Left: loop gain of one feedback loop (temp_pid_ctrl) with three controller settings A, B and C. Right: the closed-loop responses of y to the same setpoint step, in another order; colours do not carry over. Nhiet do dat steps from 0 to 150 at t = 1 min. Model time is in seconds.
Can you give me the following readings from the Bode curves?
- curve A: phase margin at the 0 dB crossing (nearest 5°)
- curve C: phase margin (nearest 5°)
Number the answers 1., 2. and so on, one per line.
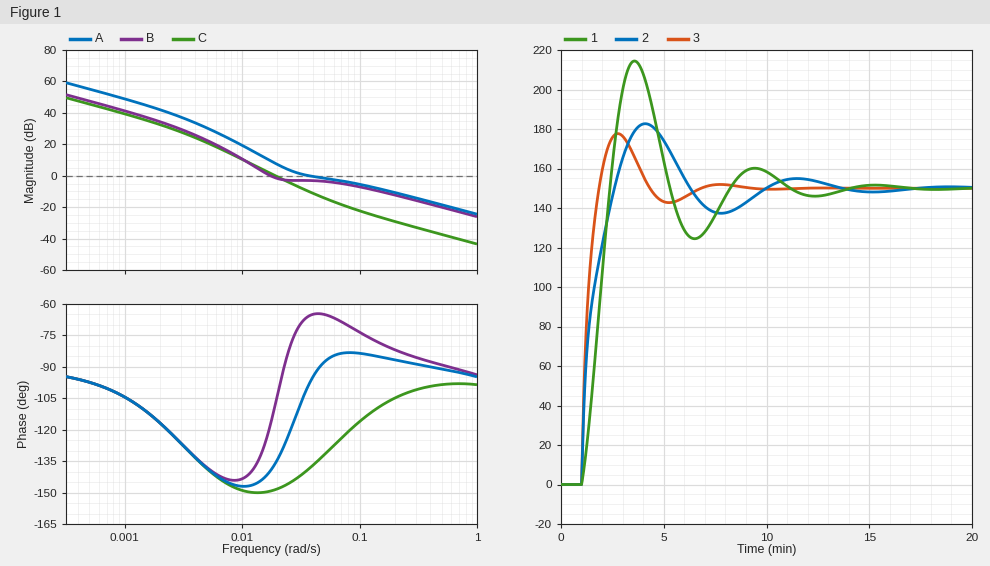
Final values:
1. 80°
2. 30°
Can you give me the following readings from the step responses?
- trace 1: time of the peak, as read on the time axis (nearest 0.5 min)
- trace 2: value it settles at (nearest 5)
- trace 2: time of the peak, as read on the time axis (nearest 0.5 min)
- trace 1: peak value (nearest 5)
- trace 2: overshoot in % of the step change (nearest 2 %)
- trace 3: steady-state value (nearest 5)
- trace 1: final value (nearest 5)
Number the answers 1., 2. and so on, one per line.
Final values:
1. 3.5 min
2. 150
3. 4.0 min
4. 215
5. 22 %
6. 150
7. 150
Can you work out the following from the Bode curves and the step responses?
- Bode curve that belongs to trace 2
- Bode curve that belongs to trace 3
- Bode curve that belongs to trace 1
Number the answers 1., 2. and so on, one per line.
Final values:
1. B
2. A
3. C
